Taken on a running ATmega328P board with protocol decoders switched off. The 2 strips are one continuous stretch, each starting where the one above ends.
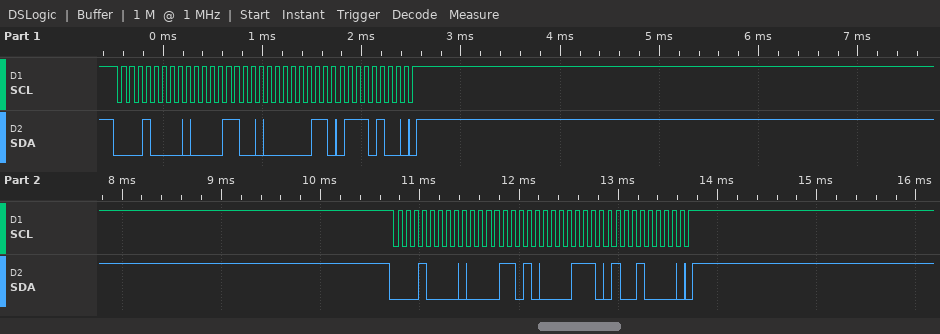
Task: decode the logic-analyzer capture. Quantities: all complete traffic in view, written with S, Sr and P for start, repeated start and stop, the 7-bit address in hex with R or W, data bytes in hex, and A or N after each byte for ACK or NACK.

S 08W A 0C A 03 A 74 A P S 08W A 0D A 0E A 90 A P
